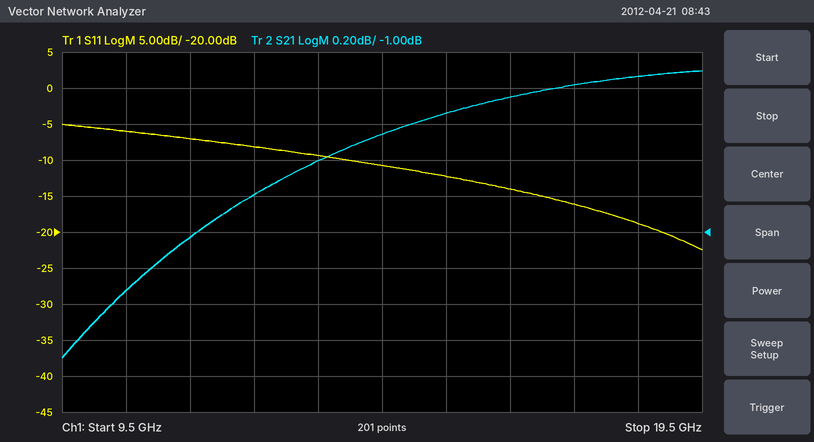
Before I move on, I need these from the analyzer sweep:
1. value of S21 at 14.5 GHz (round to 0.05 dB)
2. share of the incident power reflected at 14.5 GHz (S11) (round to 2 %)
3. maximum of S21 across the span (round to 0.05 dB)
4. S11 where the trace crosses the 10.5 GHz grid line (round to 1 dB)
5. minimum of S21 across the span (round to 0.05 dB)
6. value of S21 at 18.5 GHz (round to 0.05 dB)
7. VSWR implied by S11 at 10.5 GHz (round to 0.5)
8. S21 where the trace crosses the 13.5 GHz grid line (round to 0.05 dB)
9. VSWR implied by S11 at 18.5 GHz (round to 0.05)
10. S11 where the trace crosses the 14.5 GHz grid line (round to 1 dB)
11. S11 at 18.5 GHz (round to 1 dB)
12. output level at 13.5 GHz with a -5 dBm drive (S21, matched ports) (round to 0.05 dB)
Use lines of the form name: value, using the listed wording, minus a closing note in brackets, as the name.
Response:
value of S21 at 14.5 GHz: -0.45 dB
share of the incident power reflected at 14.5 GHz (S11): 8 %
maximum of S21 across the span: -0.10 dB
S11 where the trace crosses the 10.5 GHz grid line: -6 dB
minimum of S21 across the span: -1.70 dB
value of S21 at 18.5 GHz: -0.15 dB
VSWR implied by S11 at 10.5 GHz: 3.0
S21 where the trace crosses the 13.5 GHz grid line: -0.60 dB
VSWR implied by S11 at 18.5 GHz: 1.25
S11 where the trace crosses the 14.5 GHz grid line: -11 dB
S11 at 18.5 GHz: -19 dB
output level at 13.5 GHz with a -5 dBm drive (S21, matched ports): -5.60 dBm
